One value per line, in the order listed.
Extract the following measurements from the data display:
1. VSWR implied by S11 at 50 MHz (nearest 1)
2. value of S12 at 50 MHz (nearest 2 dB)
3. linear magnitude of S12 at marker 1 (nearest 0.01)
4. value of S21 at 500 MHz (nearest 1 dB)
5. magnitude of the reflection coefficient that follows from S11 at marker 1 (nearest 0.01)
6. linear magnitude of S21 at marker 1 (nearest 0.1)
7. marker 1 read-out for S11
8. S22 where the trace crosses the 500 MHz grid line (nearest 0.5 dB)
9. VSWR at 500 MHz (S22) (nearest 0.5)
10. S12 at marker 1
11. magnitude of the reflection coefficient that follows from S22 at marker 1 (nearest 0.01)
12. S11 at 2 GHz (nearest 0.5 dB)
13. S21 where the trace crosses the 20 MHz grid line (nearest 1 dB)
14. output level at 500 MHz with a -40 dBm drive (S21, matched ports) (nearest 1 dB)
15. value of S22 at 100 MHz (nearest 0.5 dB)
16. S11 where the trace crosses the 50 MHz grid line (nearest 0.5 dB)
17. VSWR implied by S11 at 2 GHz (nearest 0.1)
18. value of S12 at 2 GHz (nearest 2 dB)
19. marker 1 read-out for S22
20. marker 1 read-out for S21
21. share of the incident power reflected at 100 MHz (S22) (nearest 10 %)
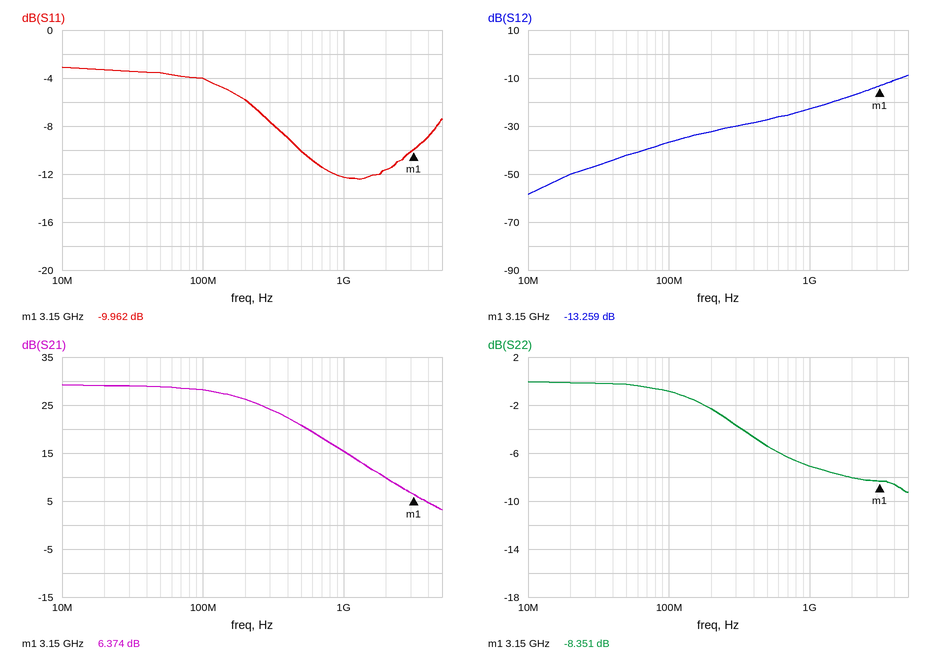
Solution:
5
-42 dB
0.22
21 dB
0.32
2.1
-9.962 dB
-5.5 dB
3.5
-13.259 dB
0.38
-11.5 dB
29 dB
-19 dBm
-1.0 dB
-3.5 dB
1.7
-18 dB
-8.351 dB
6.374 dB
80 %
